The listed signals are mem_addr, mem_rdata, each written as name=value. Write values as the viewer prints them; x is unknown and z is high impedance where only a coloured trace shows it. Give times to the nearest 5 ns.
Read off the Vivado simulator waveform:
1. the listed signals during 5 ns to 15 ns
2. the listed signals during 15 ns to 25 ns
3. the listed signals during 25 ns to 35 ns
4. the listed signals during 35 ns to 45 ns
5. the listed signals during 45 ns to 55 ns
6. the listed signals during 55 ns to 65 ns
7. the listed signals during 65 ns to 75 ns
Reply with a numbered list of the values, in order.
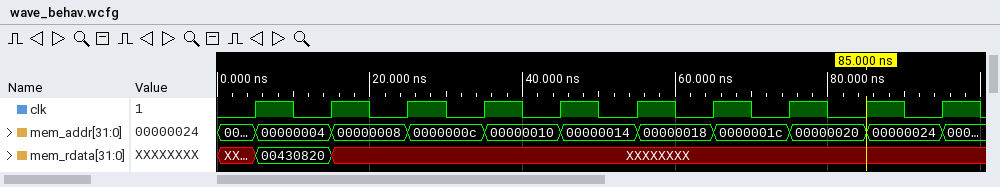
1. mem_addr=00000004, mem_rdata=00430820
2. mem_addr=00000008, mem_rdata=XXXXXXXX
3. mem_addr=0000000c, mem_rdata=XXXXXXXX
4. mem_addr=00000010, mem_rdata=XXXXXXXX
5. mem_addr=00000014, mem_rdata=XXXXXXXX
6. mem_addr=00000018, mem_rdata=XXXXXXXX
7. mem_addr=0000001c, mem_rdata=XXXXXXXX
